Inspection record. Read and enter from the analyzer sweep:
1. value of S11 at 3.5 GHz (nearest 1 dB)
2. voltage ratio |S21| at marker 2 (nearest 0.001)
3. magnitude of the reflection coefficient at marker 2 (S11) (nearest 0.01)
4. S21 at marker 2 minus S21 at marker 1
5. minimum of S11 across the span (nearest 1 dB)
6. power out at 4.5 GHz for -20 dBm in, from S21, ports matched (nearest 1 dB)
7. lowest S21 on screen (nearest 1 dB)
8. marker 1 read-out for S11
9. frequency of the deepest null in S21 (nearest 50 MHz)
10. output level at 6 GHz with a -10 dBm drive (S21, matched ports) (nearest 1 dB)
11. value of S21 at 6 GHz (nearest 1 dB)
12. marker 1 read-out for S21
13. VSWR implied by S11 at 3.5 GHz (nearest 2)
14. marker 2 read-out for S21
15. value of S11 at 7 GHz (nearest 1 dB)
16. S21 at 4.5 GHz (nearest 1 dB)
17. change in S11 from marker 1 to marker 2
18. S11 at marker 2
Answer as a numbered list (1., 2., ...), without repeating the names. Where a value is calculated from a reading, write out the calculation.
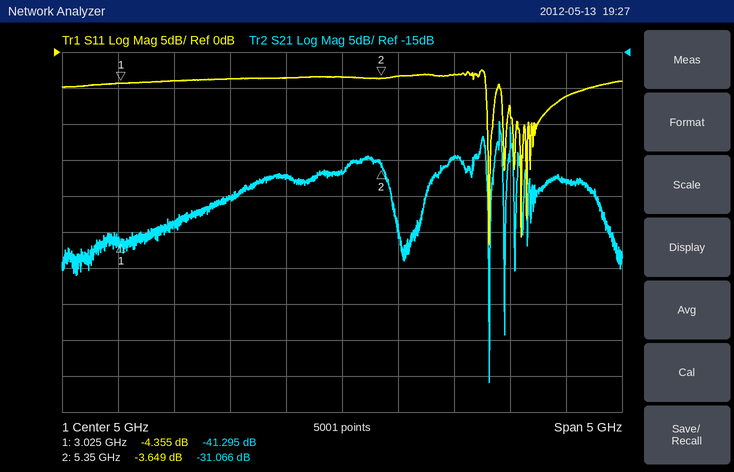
1. -4 dB
2. 10^(-31.066/20) ≈ 0.028
3. 10^(-3.649/20) ≈ 0.66
4. -31.066 − (-41.295) = 10.229 dB
5. -27 dB
6. -20 dBm + (-32 dB) = -52 dBm
7. -61 dB
8. -4.355 dB
9. 6.30 GHz
10. -10 dBm + (-30 dB) = -40 dBm
11. -30 dB
12. -41.295 dB
13. |Γ| = 10^(-4/20) = 0.6310; VSWR = (1 + 0.6310)/(1 − 0.6310) ≈ 4
14. -31.066 dB
15. -6 dB
16. -32 dB
17. -3.649 − (-4.355) = 0.706 dB
18. -3.649 dB
